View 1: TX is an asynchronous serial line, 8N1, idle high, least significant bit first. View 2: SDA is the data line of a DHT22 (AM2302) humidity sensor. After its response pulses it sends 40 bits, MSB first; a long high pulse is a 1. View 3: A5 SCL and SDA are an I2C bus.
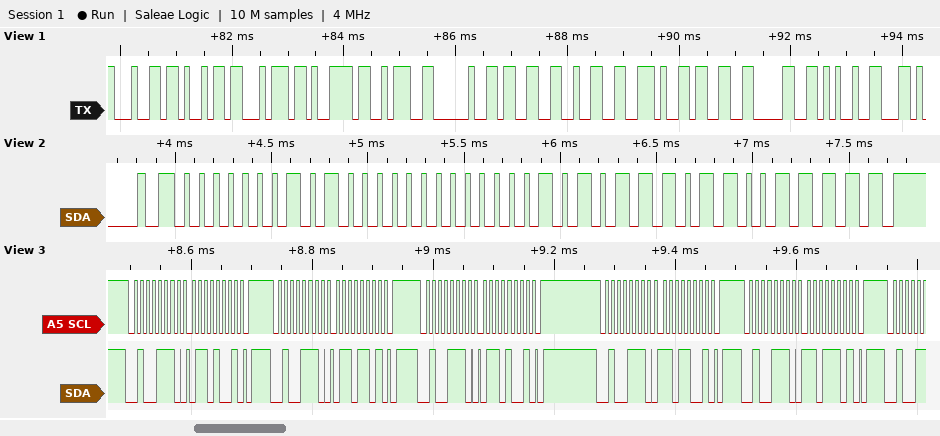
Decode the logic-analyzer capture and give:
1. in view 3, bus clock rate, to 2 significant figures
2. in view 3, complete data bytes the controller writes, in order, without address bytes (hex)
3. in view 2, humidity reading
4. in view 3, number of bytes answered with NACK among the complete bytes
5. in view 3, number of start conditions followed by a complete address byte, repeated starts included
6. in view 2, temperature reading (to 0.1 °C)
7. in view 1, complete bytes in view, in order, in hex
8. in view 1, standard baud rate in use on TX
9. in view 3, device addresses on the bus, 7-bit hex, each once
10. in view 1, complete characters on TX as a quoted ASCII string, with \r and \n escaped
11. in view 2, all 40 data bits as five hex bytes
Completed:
100 kHz
69 6D 69 D9 DD
32.0 %
0
5
34.9 °C
64 69 74 79 3A 20 33 32 2E 33 30 25
9600 baud
0x27
"dity: 32.30%"
01 40 01 5D 9F
